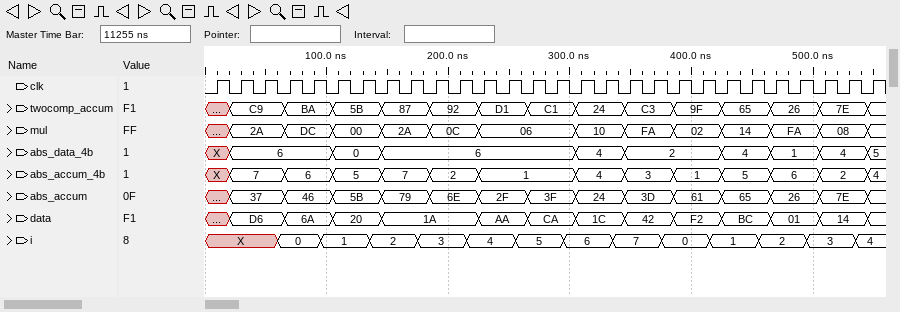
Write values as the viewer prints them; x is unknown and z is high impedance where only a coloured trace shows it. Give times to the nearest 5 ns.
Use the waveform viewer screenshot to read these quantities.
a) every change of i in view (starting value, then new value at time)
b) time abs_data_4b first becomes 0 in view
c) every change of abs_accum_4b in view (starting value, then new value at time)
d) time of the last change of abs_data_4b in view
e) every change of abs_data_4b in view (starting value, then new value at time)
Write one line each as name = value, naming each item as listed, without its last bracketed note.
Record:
every change of i in view = X, 0 at 60 ns, 1 at 95 ns, 2 at 135 ns, 3 at 175 ns, 4 at 215 ns, 5 at 255 ns, 6 at 295 ns, 7 at 335 ns, 0 at 375 ns, 1 at 415 ns, 2 at 455 ns, 3 at 495 ns, 4 at 535 ns
time abs_data_4b first becomes 0 in view = 105 ns
every change of abs_accum_4b in view = X, 7 at 20 ns, 6 at 65 ns, 5 at 105 ns, 7 at 145 ns, 2 at 185 ns, 1 at 225 ns, 4 at 305 ns, 3 at 345 ns, 1 at 385 ns, 5 at 425 ns, 6 at 465 ns, 2 at 505 ns, 4 at 545 ns
time of the last change of abs_data_4b in view = 545 ns
every change of abs_data_4b in view = X, 6 at 20 ns, 0 at 105 ns, 6 at 145 ns, 4 at 305 ns, 2 at 345 ns, 4 at 425 ns, 1 at 465 ns, 4 at 505 ns, 5 at 545 ns
